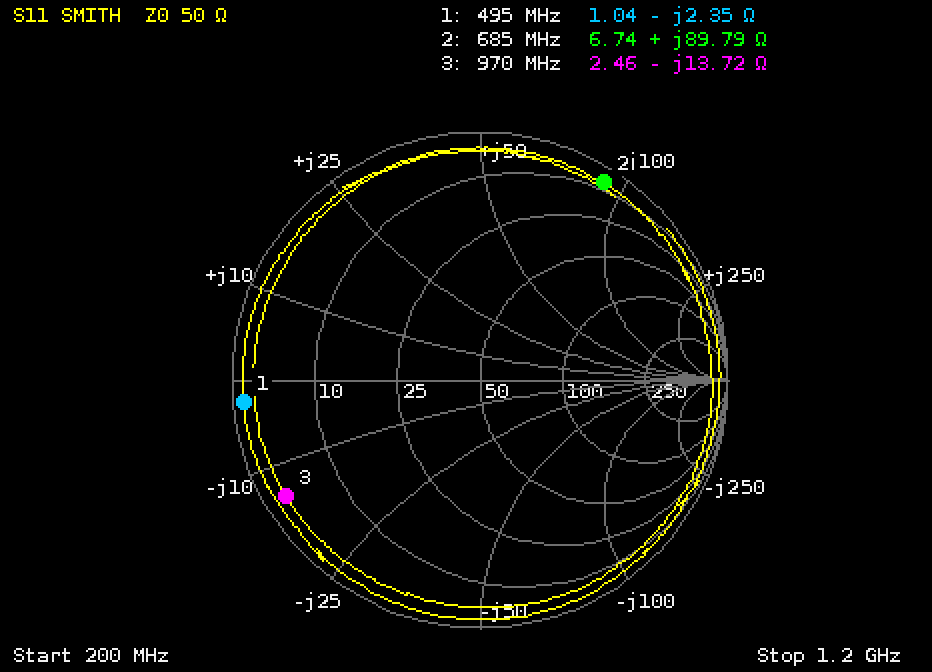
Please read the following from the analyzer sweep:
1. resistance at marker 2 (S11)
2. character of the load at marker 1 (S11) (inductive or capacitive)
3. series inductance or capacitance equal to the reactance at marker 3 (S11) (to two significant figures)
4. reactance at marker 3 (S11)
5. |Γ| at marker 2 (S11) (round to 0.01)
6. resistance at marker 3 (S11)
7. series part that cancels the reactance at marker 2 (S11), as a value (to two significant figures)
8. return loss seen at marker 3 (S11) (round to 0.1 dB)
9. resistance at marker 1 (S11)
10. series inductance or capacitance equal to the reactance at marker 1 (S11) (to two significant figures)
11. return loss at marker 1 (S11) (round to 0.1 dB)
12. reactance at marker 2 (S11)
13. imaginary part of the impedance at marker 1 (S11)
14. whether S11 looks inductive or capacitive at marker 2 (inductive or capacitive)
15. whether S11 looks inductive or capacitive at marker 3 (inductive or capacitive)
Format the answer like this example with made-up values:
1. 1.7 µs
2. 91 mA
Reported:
1. 6.74 Ω
2. capacitive
3. 12 pF
4. -13.72 Ω
5. 0.94
6. 2.46 Ω
7. 2.6 pF
8. 0.8 dB
9. 1.04 Ω
10. 140 pF
11. 0.4 dB
12. +89.79 Ω
13. -2.35 Ω
14. inductive
15. capacitive
